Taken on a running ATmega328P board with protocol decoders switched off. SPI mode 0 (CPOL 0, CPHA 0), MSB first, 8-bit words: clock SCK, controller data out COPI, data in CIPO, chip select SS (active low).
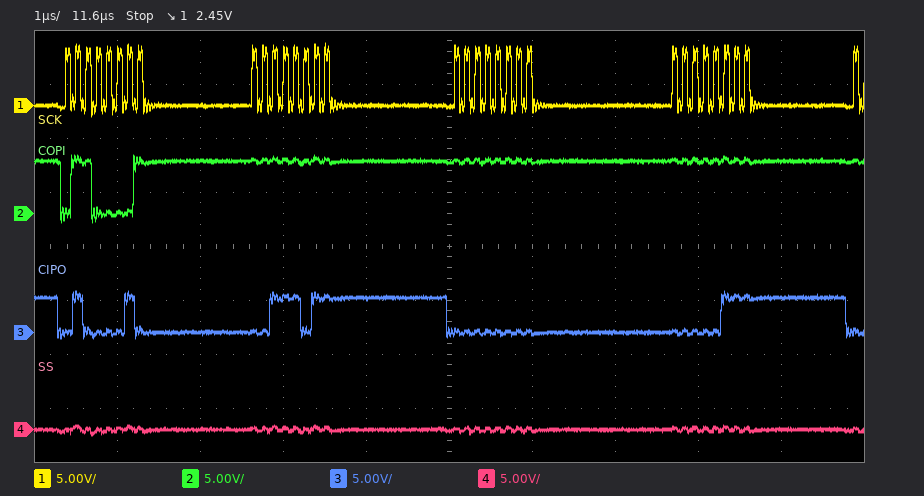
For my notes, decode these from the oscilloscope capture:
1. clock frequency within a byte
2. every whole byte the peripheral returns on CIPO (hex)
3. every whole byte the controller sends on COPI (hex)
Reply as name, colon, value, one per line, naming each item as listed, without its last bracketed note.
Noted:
clock frequency within a byte: 8 MHz
every whole byte the peripheral returns on CIPO: 0x42 0x3B 0x00 0x07
every whole byte the controller sends on COPI: 0x61 0xFF 0xFF 0xFF
